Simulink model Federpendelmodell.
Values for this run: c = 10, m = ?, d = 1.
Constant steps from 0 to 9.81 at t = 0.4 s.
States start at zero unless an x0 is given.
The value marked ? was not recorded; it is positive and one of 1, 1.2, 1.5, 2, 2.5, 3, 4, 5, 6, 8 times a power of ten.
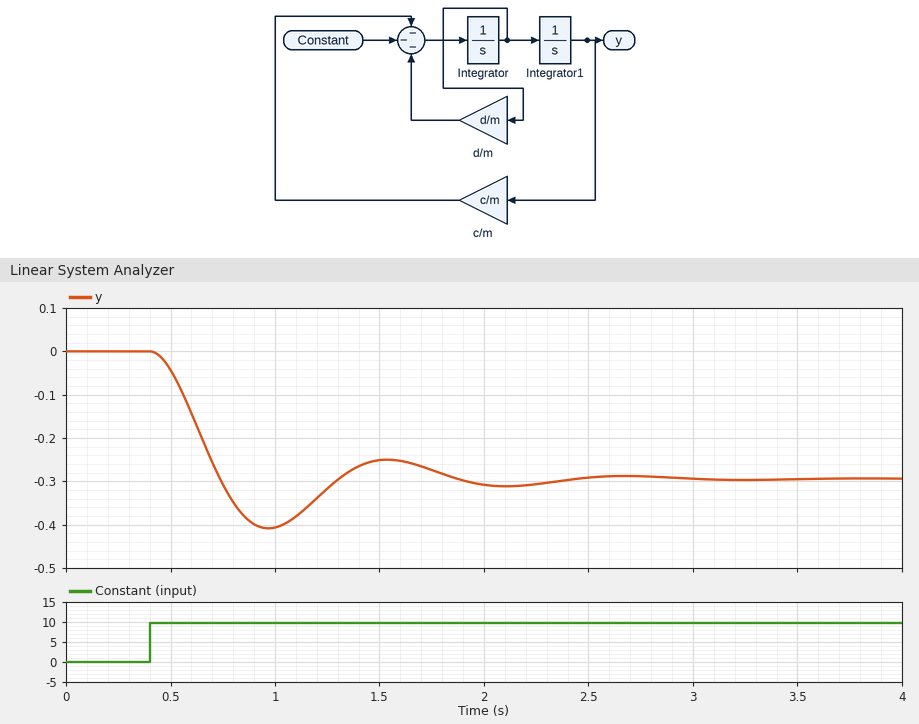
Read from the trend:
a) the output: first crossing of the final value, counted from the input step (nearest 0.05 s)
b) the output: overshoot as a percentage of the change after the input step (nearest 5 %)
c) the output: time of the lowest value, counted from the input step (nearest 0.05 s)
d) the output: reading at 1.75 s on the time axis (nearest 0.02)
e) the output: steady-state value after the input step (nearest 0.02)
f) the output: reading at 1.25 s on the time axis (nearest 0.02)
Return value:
0.35 s
40 %
0.55 s
-0.28
-0.30
-0.32
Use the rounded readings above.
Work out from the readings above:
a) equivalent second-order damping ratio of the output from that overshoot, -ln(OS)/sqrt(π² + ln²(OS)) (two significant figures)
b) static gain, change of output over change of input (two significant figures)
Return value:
0.28
-0.031
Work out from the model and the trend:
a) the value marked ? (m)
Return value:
0.3
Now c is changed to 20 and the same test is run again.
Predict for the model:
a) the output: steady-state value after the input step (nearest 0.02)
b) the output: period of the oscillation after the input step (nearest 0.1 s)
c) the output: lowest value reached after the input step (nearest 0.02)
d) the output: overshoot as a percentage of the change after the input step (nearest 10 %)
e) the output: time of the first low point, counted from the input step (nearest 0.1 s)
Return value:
-0.14
0.8 s
-0.22
50 %
0.4 s
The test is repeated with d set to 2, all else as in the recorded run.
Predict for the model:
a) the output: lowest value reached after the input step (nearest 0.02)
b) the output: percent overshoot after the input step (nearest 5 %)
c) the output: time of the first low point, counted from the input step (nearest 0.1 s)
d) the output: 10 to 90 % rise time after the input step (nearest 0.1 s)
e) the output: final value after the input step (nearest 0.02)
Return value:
-0.32
10 %
0.7 s
0.3 s
-0.30
